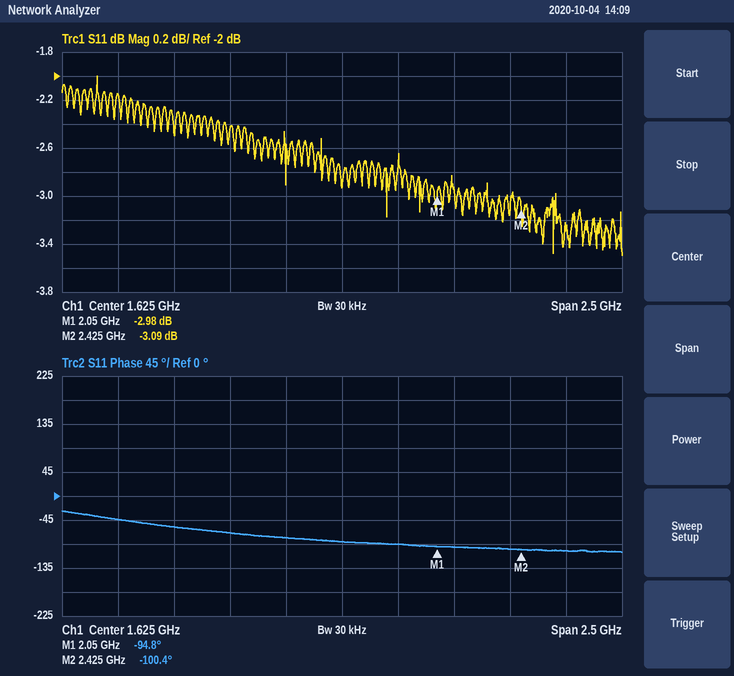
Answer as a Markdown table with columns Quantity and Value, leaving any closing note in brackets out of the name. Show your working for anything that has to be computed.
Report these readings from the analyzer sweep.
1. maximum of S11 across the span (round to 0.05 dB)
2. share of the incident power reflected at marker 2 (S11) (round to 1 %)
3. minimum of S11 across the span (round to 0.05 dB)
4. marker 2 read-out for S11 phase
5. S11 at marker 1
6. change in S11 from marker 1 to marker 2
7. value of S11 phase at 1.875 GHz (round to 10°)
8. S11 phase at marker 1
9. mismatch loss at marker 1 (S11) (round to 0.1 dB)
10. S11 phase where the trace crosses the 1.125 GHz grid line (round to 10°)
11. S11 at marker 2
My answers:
| Quantity | Value |
|---|---|
| maximum of S11 across the span | -2.00 dB |
| share of the incident power reflected at marker 2 (S11) | 10^(-3.09/10) ≈ 49 % |
| minimum of S11 across the span | -3.50 dB |
| marker 2 read-out for S11 phase | -100.4° |
| S11 at marker 1 | -2.98 dB |
| change in S11 from marker 1 to marker 2 | -3.09 − (-2.98) = -0.11 dB |
| value of S11 phase at 1.875 GHz | -90° |
| S11 phase at marker 1 | -94.8° |
| mismatch loss at marker 1 (S11) | −10 log10(1 − 10^(-2.98/10)) ≈ 3.0 dB |
| S11 phase where the trace crosses the 1.125 GHz grid line | -70° |
| S11 at marker 2 | -3.09 dB |
